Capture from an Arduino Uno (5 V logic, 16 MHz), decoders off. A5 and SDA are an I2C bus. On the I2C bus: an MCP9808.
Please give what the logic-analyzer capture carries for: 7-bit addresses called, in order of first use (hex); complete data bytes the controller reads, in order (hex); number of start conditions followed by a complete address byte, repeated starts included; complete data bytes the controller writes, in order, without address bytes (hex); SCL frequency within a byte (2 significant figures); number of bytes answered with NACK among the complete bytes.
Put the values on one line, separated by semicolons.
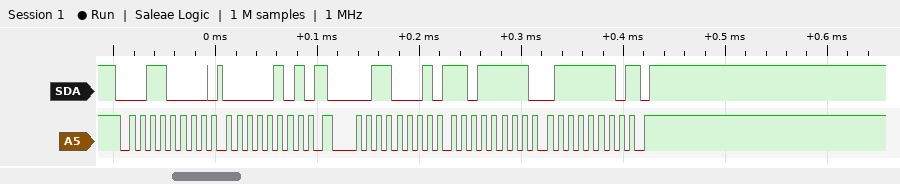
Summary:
0x18; DF 7E; 2; 05; 100 kHz; 1
